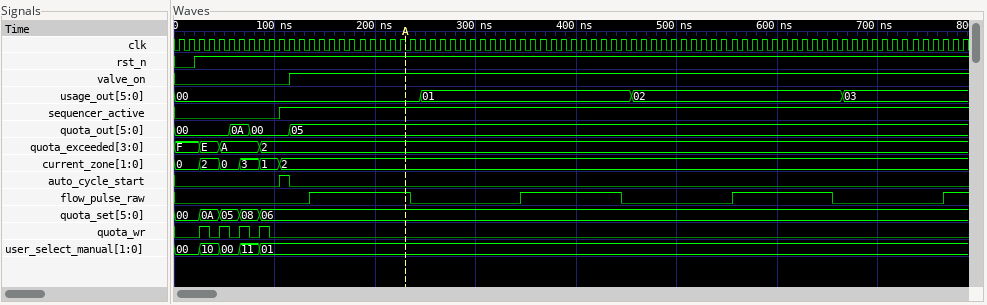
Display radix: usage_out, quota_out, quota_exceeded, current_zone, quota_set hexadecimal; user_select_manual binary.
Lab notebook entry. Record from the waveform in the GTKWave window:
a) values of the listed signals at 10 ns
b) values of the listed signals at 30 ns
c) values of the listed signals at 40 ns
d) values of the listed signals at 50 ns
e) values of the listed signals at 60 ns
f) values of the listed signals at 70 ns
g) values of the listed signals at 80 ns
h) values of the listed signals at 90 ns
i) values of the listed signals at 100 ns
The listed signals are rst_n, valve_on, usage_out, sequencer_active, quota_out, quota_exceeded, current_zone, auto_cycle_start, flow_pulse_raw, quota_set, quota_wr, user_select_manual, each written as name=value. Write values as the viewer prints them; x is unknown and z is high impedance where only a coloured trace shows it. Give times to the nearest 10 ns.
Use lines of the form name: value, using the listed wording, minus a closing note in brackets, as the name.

values of the listed signals at 10 ns: rst_n=0, valve_on=0, usage_out=00, sequencer_active=0, quota_out=00, quota_exceeded=F, current_zone=0, auto_cycle_start=0, flow_pulse_raw=0, quota_set=00, quota_wr=0, user_select_manual=00
values of the listed signals at 30 ns: rst_n=1, valve_on=0, usage_out=00, sequencer_active=0, quota_out=00, quota_exceeded=E, current_zone=2, auto_cycle_start=0, flow_pulse_raw=0, quota_set=0A, quota_wr=1, user_select_manual=10
values of the listed signals at 40 ns: rst_n=1, valve_on=0, usage_out=00, sequencer_active=0, quota_out=00, quota_exceeded=E, current_zone=2, auto_cycle_start=0, flow_pulse_raw=0, quota_set=0A, quota_wr=0, user_select_manual=10
values of the listed signals at 50 ns: rst_n=1, valve_on=0, usage_out=00, sequencer_active=0, quota_out=00, quota_exceeded=A, current_zone=0, auto_cycle_start=0, flow_pulse_raw=0, quota_set=05, quota_wr=1, user_select_manual=00
values of the listed signals at 60 ns: rst_n=1, valve_on=0, usage_out=00, sequencer_active=0, quota_out=0A, quota_exceeded=A, current_zone=0, auto_cycle_start=0, flow_pulse_raw=0, quota_set=05, quota_wr=0, user_select_manual=00
values of the listed signals at 70 ns: rst_n=1, valve_on=0, usage_out=00, sequencer_active=0, quota_out=0A, quota_exceeded=A, current_zone=3, auto_cycle_start=0, flow_pulse_raw=0, quota_set=08, quota_wr=1, user_select_manual=11
values of the listed signals at 80 ns: rst_n=1, valve_on=0, usage_out=00, sequencer_active=0, quota_out=00, quota_exceeded=A, current_zone=3, auto_cycle_start=0, flow_pulse_raw=0, quota_set=08, quota_wr=0, user_select_manual=11
values of the listed signals at 90 ns: rst_n=1, valve_on=0, usage_out=00, sequencer_active=0, quota_out=00, quota_exceeded=2, current_zone=1, auto_cycle_start=0, flow_pulse_raw=0, quota_set=06, quota_wr=1, user_select_manual=01
values of the listed signals at 100 ns: rst_n=1, valve_on=0, usage_out=00, sequencer_active=0, quota_out=00, quota_exceeded=2, current_zone=1, auto_cycle_start=0, flow_pulse_raw=0, quota_set=06, quota_wr=0, user_select_manual=01
